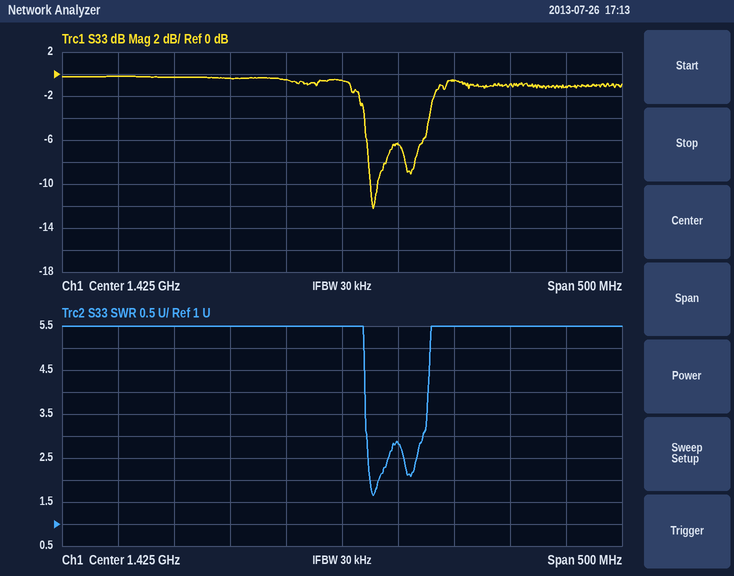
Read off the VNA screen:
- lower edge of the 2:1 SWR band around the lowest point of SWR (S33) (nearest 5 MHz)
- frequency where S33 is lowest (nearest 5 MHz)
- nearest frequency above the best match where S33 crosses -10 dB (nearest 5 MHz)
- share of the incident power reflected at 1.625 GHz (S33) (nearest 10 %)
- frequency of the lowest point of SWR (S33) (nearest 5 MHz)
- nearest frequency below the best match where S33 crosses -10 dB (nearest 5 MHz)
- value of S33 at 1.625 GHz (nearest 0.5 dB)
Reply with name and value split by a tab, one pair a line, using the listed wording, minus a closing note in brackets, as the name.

lower edge of the 2:1 SWR band around the lowest point of SWR (S33)	1.450 GHz
frequency where S33 is lowest	1.455 GHz
nearest frequency above the best match where S33 crosses -10 dB	1.455 GHz
share of the incident power reflected at 1.625 GHz (S33)	80 %
frequency of the lowest point of SWR (S33)	1.455 GHz
nearest frequency below the best match where S33 crosses -10 dB	1.450 GHz
value of S33 at 1.625 GHz	-1.0 dB
